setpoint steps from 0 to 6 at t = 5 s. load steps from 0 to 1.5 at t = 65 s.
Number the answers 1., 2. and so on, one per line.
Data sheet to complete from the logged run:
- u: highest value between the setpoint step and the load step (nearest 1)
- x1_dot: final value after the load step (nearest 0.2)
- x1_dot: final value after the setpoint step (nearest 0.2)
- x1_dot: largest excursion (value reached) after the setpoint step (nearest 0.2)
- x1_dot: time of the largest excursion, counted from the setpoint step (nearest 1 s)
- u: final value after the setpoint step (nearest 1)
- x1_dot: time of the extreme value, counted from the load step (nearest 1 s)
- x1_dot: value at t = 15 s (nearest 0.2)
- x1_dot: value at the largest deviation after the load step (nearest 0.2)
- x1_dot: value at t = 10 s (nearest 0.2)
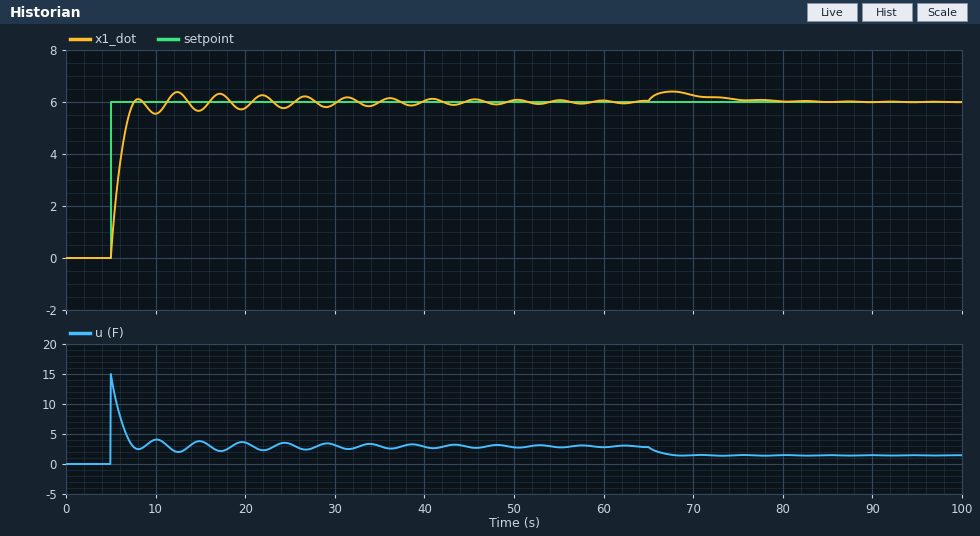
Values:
1. 15
2. 6.0
3. 6.0
4. 6.4
5. 7 s
6. 3
7. 3 s
8. 5.6
9. 6.4
10. 5.6
